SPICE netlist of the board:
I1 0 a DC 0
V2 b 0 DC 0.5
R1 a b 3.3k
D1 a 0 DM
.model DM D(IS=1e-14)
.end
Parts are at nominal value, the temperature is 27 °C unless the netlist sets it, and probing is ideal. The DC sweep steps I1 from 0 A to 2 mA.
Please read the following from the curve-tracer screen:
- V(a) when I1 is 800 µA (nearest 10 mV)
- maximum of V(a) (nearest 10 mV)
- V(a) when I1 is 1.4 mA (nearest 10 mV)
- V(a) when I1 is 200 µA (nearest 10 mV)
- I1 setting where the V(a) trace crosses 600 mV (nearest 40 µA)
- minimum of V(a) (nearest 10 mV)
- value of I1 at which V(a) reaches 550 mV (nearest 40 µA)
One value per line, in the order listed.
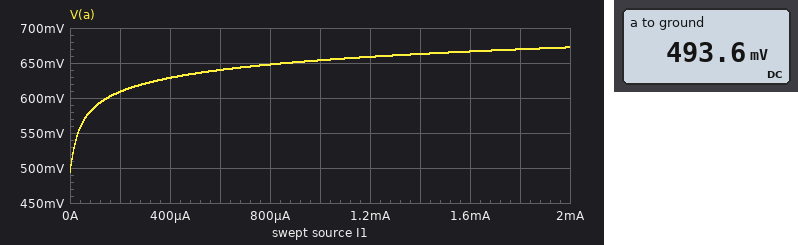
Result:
650 mV
670 mV
660 mV
610 mV
160 µA
490 mV
40 µA
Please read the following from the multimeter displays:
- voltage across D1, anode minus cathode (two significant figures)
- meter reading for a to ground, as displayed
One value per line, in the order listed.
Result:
490 mV
493.6 mV
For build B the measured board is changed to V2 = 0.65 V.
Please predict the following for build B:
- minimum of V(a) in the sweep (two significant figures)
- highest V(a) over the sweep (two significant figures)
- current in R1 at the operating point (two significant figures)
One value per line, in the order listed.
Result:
560 mV
670 mV
27 µA
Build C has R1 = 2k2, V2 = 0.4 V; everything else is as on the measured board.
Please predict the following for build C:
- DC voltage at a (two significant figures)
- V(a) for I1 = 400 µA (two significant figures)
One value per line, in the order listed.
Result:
400 mV
620 mV
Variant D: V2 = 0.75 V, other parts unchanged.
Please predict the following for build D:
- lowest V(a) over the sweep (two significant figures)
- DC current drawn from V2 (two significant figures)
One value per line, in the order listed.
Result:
580 mV
52 µA
